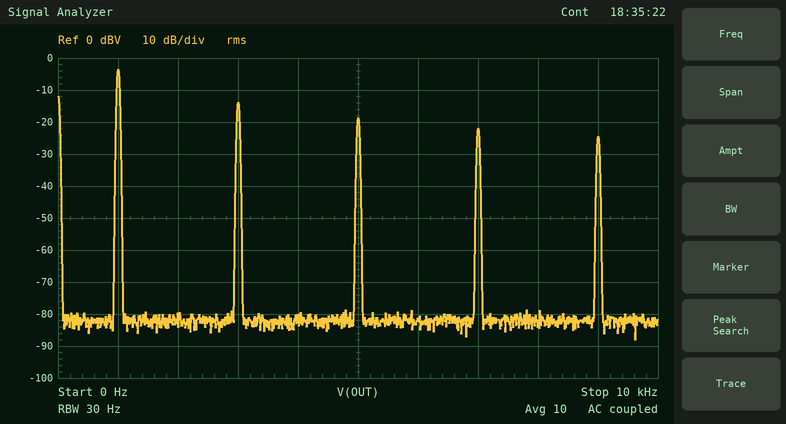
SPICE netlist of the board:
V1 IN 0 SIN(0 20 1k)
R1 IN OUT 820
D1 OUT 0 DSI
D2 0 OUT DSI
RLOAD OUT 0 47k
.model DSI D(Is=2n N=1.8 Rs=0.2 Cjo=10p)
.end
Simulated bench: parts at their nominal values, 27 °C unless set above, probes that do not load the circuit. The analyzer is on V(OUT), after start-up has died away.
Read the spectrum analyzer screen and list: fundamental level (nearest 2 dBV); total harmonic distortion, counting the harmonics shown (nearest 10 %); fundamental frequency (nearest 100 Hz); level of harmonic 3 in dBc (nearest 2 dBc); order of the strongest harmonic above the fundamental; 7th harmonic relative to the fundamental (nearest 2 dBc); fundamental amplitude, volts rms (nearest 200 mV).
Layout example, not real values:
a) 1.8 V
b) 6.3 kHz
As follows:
a) -4 dBV
b) 40 %
c) 1.0 kHz
d) -10 dBc
e) 3
f) -18 dBc
g) 600 mV
